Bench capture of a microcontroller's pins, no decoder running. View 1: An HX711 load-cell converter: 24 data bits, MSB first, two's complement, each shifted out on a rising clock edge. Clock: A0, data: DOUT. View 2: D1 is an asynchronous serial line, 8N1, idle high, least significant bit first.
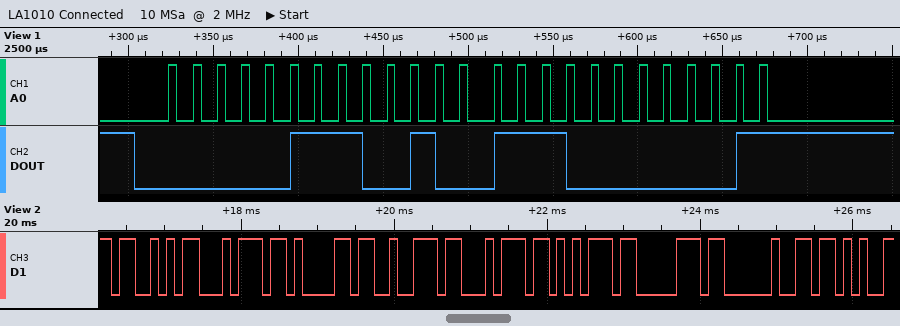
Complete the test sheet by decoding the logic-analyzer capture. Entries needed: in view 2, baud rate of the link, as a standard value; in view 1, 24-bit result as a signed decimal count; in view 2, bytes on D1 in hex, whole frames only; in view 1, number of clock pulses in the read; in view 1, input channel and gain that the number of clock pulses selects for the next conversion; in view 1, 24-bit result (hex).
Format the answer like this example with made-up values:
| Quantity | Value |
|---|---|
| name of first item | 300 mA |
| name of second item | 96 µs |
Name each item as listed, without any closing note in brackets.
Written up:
| Quantity | Value |
|---|---|
| in view 2, baud rate of the link, as a standard value | 9600 baud |
| in view 1, 24-bit result as a signed decimal count | 468737 |
| in view 2, bytes on D1 in hex, whole frames only | 53 74 61 72 74 75 70 20 2B |
| in view 1, number of clock pulses in the read | 25 |
| in view 1, input channel and gain that the number of clock pulses selects for the next conversion | channel A, gain 128 |
| in view 1, 24-bit result | 0x072701 |
